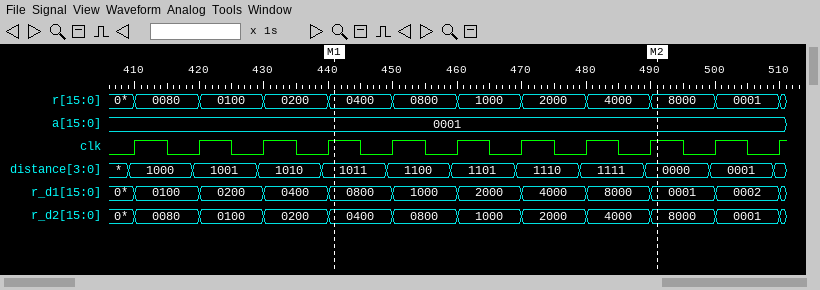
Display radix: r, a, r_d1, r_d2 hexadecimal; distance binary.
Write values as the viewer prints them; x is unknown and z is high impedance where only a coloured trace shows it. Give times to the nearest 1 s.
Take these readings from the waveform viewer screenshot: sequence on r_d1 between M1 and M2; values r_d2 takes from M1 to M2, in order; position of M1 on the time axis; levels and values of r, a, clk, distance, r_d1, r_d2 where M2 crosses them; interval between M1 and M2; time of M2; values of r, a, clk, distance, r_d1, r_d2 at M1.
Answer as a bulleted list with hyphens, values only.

- 0800, 1000, 2000, 4000, 8000, 0001
- 0400, 0800, 1000, 2000, 4000, 8000
- 441 s
- r=8000, a=0001, clk=1, distance=0000, r_d1=0001, r_d2=8000
- 50 s
- 491 s
- r=0400, a=0001, clk=1, distance=1011, r_d1=0800, r_d2=0400
